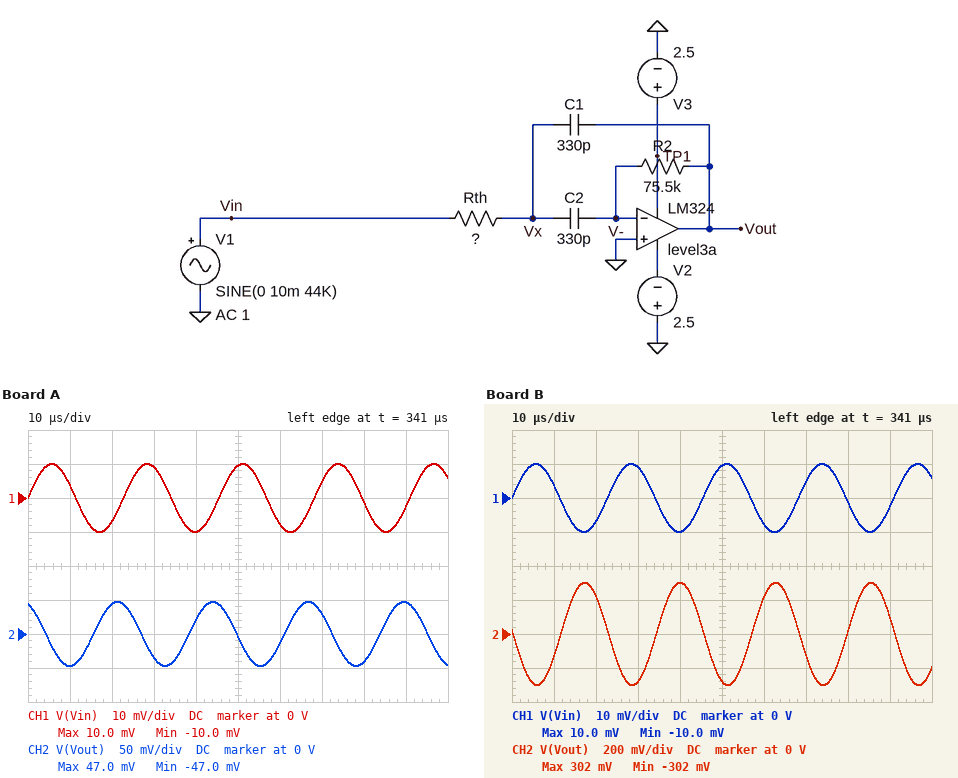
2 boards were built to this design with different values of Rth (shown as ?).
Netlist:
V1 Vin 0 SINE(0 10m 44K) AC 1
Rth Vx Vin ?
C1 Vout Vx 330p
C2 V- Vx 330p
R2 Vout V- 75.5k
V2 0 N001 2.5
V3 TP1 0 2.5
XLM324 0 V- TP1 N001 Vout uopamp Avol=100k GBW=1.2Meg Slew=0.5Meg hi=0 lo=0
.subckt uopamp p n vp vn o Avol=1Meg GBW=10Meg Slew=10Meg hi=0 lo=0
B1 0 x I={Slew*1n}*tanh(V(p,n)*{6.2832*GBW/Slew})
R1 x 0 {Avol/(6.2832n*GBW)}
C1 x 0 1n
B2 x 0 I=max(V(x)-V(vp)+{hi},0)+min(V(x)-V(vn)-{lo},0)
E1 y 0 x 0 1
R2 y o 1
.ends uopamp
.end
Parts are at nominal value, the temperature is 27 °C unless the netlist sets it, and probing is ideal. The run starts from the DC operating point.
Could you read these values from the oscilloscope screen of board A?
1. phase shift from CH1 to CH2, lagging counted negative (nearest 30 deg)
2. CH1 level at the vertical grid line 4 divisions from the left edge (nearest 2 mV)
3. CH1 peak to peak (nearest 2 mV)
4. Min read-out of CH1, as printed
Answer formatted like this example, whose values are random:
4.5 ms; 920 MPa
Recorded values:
120 deg; -10 mV; 20 mV; -10.0 mV
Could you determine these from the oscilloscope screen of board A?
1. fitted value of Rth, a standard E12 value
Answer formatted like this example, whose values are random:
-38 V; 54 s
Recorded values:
3.3 kΩ
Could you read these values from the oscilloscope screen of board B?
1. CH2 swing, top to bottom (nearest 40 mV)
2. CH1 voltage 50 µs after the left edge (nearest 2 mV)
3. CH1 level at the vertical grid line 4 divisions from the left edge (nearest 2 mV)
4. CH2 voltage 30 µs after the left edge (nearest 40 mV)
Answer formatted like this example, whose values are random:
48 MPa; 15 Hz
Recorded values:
600 mV; 10 mV; -10 mV; -280 mV
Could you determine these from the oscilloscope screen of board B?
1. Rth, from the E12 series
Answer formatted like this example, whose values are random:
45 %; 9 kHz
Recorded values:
1.2 kΩ
